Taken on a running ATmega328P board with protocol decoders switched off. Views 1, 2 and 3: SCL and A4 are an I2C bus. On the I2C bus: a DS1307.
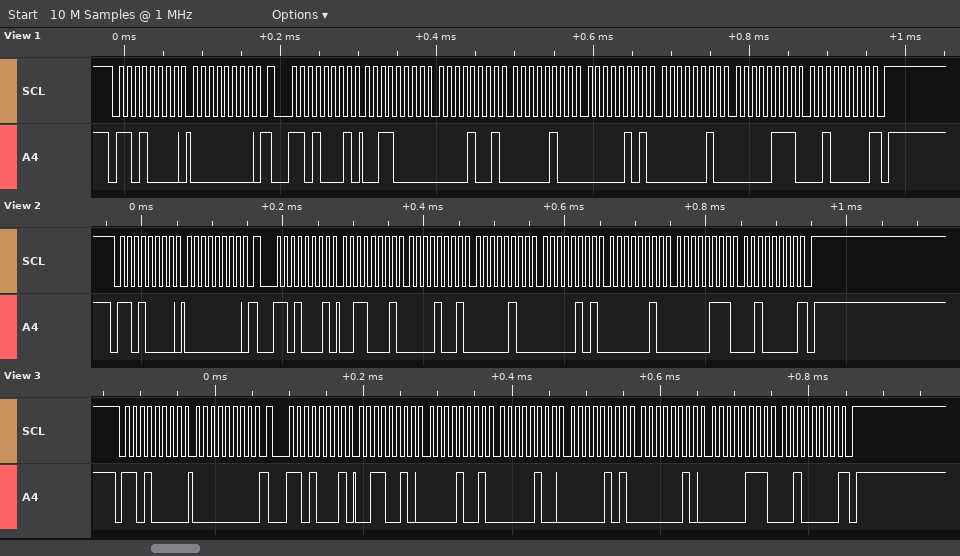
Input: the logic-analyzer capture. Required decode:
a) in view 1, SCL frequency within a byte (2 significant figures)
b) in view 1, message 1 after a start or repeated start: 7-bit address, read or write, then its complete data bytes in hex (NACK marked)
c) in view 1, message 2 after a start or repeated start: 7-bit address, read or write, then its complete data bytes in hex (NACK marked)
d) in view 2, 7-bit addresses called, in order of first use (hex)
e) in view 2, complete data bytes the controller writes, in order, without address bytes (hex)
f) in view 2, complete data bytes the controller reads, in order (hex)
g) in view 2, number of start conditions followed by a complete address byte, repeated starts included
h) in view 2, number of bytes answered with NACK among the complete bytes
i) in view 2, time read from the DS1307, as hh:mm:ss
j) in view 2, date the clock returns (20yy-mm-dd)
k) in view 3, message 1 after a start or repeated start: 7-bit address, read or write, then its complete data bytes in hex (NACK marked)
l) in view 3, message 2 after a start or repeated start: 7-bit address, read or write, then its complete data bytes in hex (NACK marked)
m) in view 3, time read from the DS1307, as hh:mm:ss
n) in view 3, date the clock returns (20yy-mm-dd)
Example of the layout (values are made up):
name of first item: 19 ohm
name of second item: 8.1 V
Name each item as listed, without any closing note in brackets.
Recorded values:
in view 1, SCL frequency within a byte: 100 kHz
in view 1, message 1 after a start or repeated start: 7-bit address, read or write, then its complete data bytes in hex: 0x68 write: 00
in view 1, message 2 after a start or repeated start: 7-bit address, read or write, then its complete data bytes in hex: 0x68 read: 30 09 04 05 02 07 20 NACK
in view 2, 7-bit addresses called, in order of first use: 0x68
in view 2, complete data bytes the controller writes, in order, without address bytes: 00
in view 2, complete data bytes the controller reads, in order: 31 09 04 05 02 07 20
in view 2, number of start conditions followed by a complete address byte, repeated starts included: 2
in view 2, number of bytes answered with NACK among the complete bytes: 1
in view 2, time read from the DS1307, as hh:mm:ss: 04:09:31
in view 2, date the clock returns: 2020-07-02
in view 3, message 1 after a start or repeated start: 7-bit address, read or write, then its complete data bytes in hex: 0x68 write: 00
in view 3, message 2 after a start or repeated start: 7-bit address, read or write, then its complete data bytes in hex: 0x68 read: 32 09 04 05 02 07 20 NACK
in view 3, time read from the DS1307, as hh:mm:ss: 04:09:32
in view 3, date the clock returns: 2020-07-02
